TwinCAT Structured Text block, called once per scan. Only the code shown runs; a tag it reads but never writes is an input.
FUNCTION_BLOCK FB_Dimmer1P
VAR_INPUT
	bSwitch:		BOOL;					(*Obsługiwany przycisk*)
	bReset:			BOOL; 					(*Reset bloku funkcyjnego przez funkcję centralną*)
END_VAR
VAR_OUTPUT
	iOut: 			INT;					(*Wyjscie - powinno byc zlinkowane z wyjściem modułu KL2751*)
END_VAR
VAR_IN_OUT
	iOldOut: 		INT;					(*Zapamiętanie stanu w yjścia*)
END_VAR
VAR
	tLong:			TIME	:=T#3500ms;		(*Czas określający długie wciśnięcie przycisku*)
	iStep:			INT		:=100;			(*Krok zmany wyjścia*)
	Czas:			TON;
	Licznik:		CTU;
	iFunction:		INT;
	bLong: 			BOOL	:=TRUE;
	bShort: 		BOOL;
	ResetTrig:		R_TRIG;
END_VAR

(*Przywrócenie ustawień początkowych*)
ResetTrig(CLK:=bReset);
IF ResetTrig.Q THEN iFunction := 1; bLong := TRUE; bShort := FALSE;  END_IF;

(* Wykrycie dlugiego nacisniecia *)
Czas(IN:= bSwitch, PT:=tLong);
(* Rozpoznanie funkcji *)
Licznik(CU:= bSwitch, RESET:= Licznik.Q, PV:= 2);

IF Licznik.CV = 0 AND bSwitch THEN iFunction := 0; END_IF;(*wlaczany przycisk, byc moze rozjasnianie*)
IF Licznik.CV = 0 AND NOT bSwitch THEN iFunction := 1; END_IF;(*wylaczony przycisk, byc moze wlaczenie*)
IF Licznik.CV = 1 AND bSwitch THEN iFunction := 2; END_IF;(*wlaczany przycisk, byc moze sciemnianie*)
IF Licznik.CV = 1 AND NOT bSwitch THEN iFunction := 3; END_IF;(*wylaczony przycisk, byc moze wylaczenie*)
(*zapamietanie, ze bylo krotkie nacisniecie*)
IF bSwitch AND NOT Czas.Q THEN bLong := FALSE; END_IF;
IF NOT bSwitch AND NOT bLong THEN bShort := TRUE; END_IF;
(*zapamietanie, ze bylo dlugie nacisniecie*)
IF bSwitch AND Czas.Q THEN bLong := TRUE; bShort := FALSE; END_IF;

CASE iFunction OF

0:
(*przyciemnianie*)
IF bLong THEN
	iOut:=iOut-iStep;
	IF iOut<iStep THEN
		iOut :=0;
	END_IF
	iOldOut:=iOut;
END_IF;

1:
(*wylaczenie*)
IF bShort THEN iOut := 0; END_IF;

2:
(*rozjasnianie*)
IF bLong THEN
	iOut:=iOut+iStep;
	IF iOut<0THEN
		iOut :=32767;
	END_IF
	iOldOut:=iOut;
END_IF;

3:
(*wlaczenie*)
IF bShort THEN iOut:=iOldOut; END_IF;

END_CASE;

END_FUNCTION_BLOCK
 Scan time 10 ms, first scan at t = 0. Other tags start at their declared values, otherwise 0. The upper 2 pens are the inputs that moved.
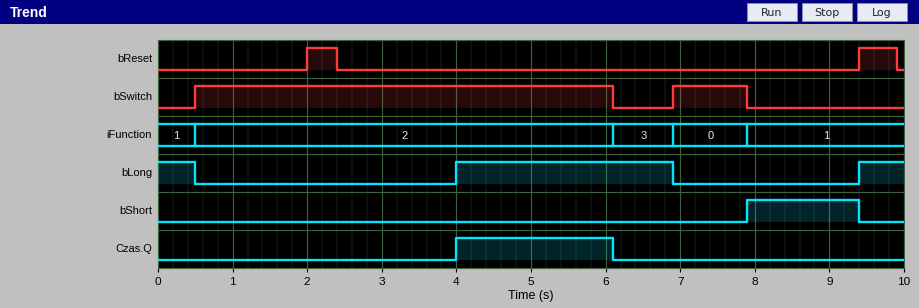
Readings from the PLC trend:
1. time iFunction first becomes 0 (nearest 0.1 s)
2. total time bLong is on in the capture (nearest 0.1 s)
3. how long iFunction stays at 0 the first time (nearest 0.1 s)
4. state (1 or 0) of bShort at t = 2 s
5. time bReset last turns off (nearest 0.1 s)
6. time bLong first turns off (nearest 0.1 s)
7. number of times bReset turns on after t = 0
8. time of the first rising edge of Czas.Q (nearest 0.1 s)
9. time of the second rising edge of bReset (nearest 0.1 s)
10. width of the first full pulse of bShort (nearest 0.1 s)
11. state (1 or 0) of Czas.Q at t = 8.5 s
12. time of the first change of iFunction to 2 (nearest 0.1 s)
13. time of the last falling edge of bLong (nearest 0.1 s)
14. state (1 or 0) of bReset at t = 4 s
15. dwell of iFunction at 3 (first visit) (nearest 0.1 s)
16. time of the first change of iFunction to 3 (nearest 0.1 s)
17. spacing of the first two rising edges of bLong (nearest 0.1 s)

6.9 s
4.0 s
1.0 s
0
9.9 s
0.5 s
2
4.0 s
9.4 s
1.5 s
0
0.5 s
6.9 s
0
0.8 s
6.1 s
5.4 s
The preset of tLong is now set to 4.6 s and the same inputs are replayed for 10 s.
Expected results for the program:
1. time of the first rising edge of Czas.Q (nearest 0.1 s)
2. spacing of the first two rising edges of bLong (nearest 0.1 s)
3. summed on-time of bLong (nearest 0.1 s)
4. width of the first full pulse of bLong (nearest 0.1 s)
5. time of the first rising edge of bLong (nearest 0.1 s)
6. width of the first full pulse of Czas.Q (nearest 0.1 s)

5.1 s
4.3 s
2.9 s
1.8 s
5.1 s
1.0 s
